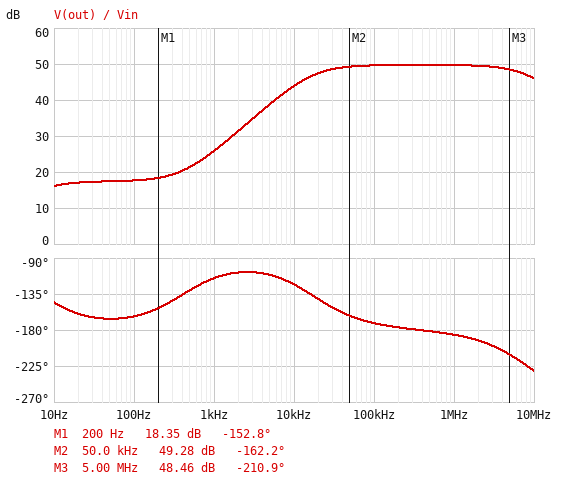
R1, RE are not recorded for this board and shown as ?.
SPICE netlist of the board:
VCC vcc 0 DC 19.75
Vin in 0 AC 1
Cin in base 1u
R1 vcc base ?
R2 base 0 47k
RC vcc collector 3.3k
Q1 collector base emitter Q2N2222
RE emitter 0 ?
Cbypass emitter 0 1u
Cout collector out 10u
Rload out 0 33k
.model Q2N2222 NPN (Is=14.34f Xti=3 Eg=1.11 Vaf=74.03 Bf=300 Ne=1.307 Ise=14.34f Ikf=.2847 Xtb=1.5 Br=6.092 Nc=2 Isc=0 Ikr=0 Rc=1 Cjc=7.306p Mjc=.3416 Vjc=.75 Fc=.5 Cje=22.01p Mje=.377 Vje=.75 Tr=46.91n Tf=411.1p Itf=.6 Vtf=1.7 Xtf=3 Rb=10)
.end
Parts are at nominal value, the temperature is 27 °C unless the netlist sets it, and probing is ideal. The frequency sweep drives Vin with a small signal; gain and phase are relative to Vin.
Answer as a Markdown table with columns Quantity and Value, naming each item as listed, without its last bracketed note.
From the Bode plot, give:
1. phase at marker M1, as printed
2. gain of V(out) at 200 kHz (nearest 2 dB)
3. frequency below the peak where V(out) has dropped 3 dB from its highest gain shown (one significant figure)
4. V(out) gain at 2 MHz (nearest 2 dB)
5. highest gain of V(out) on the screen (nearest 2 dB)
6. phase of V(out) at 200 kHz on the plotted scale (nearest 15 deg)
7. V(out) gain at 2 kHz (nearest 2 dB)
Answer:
| Quantity | Value |
|---|---|
| phase at marker M1, as printed | -152.8 deg |
| gain of V(out) at 200 kHz | 50 dB |
| frequency below the peak where V(out) has dropped 3 dB from its highest gain shown | 20 kHz |
| V(out) gain at 2 MHz | 50 dB |
| highest gain of V(out) on the screen | 50 dB |
| phase of V(out) at 200 kHz on the plotted scale | -180 deg |
| V(out) gain at 2 kHz | 32 dB |
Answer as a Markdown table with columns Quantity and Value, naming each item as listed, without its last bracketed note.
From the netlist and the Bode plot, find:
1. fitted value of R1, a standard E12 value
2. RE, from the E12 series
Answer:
| Quantity | Value |
|---|---|
| fitted value of R1, a standard E12 value | 330 kΩ |
| RE, from the E12 series | 390 Ω |
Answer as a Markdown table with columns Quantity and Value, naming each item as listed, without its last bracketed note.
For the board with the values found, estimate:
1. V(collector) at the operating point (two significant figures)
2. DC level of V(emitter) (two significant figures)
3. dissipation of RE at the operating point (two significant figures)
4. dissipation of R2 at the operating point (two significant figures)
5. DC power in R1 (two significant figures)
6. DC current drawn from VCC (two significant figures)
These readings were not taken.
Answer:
| Quantity | Value |
|---|---|
| V(collector) at the operating point | 9.9 V |
| DC level of V(emitter) | 1.2 V |
| dissipation of RE at the operating point | 3.5 mW |
| dissipation of R2 at the operating point | 72 µW |
| DC power in R1 | 970 µW |
| DC current drawn from VCC | 3.0 mA |
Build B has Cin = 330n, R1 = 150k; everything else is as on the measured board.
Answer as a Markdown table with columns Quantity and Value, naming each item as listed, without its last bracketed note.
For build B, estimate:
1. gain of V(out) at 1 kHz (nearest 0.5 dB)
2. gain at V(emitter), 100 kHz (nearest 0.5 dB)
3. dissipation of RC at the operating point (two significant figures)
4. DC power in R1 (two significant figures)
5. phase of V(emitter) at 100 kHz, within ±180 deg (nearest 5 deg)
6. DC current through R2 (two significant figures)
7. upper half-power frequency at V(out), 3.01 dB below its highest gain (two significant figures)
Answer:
| Quantity | Value |
|---|---|
| gain of V(out) at 1 kHz | 3.0 dB |
| gain at V(emitter), 100 kHz | -26.5 dB |
| dissipation of RC at the operating point | 93 mW |
| DC power in R1 | 1.9 mW |
| phase of V(emitter) at 100 kHz, within ±180 deg | -75 deg |
| DC current through R2 | 59 µA |
| upper half-power frequency at V(out), 3.01 dB below its highest gain | 1.7 MHz |
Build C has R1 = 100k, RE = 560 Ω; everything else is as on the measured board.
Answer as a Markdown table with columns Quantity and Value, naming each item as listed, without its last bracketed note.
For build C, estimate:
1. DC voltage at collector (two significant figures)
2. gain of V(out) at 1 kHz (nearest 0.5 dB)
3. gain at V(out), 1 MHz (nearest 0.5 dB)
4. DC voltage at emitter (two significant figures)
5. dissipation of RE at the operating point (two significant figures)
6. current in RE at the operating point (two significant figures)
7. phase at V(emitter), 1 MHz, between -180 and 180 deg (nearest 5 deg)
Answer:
| Quantity | Value |
|---|---|
| DC voltage at collector | 3.0 V |
| gain of V(out) at 1 kHz | 1.5 dB |
| gain at V(out), 1 MHz | 18.0 dB |
| DC voltage at emitter | 2.9 V |
| dissipation of RE at the operating point | 15 mW |
| current in RE at the operating point | 5.2 mA |
| phase at V(emitter), 1 MHz, between -180 and 180 deg | -65 deg |
